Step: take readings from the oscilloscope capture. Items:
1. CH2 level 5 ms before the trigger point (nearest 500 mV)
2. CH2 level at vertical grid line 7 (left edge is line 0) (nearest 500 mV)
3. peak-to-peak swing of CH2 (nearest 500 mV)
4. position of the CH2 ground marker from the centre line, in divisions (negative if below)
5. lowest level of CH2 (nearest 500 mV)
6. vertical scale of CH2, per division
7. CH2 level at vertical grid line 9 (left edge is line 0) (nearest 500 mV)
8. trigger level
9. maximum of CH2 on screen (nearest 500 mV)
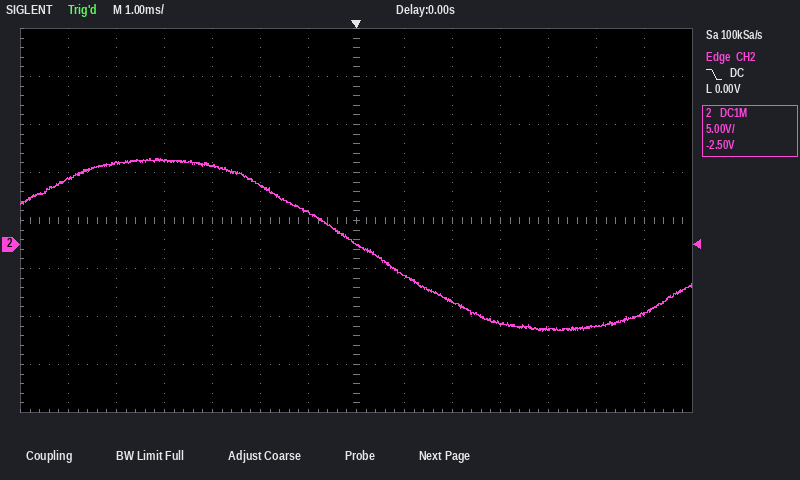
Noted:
8.5 V
0.0 V
18.0 V
-0.5 div
-9.0 V
5 V
-6.0 V
0.00 V
9.0 V
